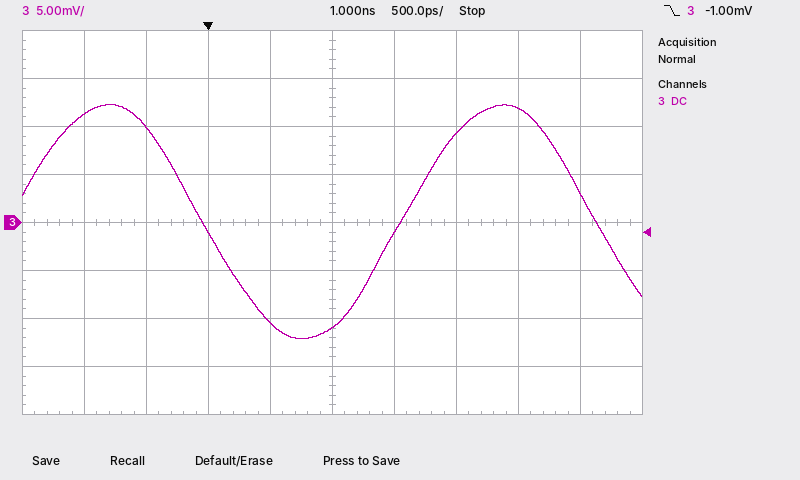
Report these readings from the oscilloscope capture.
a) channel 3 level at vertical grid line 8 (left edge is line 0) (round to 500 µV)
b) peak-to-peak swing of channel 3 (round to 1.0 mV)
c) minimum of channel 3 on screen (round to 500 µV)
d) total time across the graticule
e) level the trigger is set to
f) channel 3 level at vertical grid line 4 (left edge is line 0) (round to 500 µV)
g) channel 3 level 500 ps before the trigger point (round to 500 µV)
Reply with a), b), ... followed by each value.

a) 12.0 mV
b) 24.0 mV
c) -12.0 mV
d) 5 ns
e) -1.00 mV
f) -10.5 mV
g) 10.0 mV
